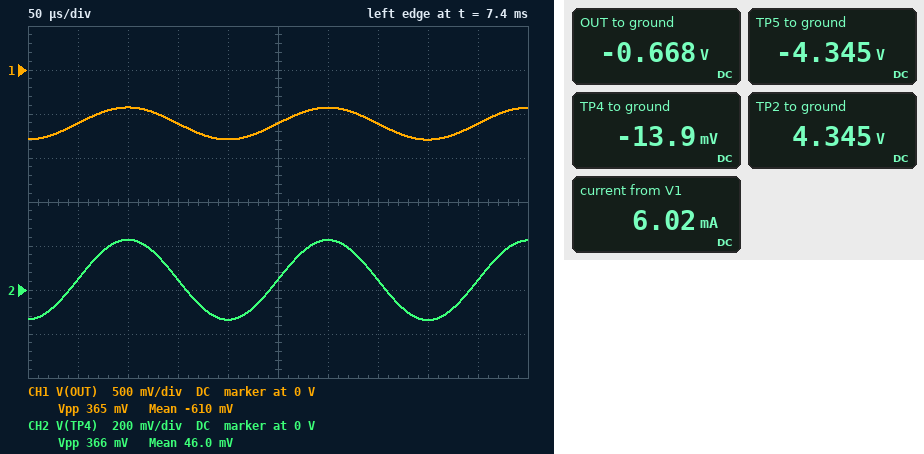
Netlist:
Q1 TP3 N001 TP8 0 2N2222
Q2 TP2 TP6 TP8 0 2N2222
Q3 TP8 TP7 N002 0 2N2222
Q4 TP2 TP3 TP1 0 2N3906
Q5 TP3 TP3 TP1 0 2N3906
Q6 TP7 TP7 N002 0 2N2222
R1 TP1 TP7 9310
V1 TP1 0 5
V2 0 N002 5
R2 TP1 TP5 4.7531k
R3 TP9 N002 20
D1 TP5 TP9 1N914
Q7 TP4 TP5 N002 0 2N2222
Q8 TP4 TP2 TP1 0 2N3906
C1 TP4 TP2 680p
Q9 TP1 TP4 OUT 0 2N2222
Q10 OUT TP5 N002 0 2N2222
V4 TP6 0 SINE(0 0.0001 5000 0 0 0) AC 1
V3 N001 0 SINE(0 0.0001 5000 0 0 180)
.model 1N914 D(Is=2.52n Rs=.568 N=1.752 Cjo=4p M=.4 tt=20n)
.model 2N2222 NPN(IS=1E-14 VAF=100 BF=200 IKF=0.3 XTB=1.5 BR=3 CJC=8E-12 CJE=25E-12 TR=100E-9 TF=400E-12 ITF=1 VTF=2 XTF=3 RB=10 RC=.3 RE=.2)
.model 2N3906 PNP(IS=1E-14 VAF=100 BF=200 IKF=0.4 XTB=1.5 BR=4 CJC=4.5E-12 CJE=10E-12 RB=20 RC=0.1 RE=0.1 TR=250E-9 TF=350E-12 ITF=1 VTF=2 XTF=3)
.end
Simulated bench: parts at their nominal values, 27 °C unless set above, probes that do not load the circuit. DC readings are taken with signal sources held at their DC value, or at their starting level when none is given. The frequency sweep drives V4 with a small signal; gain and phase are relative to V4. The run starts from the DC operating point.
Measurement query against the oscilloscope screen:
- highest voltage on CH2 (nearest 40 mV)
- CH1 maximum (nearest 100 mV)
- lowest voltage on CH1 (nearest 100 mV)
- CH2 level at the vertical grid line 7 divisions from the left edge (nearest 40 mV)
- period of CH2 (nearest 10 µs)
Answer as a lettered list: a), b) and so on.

a) 240 mV
b) -400 mV
c) -800 mV
d) 40 mV
e) 200 µs
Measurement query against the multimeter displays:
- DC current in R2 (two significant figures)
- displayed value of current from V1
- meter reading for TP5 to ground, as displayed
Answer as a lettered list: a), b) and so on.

a) 2.0 mA
b) 6.02 mA
c) -4.345 V
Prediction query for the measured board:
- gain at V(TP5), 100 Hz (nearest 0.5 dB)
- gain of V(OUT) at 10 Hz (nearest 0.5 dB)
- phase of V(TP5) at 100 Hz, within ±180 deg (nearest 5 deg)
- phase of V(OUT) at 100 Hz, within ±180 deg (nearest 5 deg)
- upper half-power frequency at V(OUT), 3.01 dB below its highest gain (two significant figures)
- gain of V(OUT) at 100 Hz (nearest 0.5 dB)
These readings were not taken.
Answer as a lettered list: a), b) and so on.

a) -39.5 dB
b) 105.0 dB
c) 5 deg
d) -75 deg
e) 23 Hz
f) 93.0 dB
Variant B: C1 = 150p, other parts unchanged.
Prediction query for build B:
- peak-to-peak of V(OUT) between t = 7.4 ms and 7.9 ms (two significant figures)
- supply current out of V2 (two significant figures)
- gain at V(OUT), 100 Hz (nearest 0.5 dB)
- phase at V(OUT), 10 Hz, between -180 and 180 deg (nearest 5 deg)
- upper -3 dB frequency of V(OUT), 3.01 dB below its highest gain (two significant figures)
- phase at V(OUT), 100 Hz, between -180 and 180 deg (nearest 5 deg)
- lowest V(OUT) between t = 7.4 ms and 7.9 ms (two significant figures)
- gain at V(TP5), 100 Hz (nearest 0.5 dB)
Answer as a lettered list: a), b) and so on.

a) 1.6 V
b) 6.0 mA
c) 103.0 dB
d) -5 deg
e) 100 Hz
f) -45 deg
g) -1.5 V
h) -29.5 dB
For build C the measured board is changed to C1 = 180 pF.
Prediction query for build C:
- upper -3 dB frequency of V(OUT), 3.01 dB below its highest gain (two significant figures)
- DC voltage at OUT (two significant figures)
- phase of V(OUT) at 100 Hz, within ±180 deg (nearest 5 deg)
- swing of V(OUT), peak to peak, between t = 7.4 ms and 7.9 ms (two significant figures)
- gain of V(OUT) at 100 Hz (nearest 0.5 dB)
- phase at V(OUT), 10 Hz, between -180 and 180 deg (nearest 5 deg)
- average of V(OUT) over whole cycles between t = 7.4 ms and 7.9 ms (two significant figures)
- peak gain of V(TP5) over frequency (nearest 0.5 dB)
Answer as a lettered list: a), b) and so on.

a) 86 Hz
b) -670 mV
c) -50 deg
d) 1.4 V
e) 102.0 dB
f) -5 deg
g) -660 mV
h) -28.0 dB
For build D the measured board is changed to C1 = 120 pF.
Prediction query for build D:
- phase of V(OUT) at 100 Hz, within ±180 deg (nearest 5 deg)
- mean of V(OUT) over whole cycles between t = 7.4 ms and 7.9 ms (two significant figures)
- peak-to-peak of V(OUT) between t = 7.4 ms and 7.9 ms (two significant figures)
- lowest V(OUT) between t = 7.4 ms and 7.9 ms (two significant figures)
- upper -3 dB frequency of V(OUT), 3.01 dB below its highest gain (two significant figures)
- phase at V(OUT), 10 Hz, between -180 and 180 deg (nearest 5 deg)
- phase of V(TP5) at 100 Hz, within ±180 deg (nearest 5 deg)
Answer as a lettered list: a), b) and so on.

a) -40 deg
b) -670 mV
c) 2.0 V
d) -1.7 V
e) 130 Hz
f) -5 deg
g) 45 deg
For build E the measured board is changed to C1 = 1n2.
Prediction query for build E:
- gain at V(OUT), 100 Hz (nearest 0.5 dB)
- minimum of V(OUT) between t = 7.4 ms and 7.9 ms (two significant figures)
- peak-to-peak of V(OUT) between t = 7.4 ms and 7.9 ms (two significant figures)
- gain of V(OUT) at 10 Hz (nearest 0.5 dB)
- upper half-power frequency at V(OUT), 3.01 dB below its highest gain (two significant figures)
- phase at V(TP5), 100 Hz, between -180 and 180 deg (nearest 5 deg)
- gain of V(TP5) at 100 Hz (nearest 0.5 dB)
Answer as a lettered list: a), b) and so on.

a) 88.0 dB
b) -720 mV
c) 210 mV
d) 104.0 dB
e) 13 Hz
f) 0 deg
g) -44.5 dB
